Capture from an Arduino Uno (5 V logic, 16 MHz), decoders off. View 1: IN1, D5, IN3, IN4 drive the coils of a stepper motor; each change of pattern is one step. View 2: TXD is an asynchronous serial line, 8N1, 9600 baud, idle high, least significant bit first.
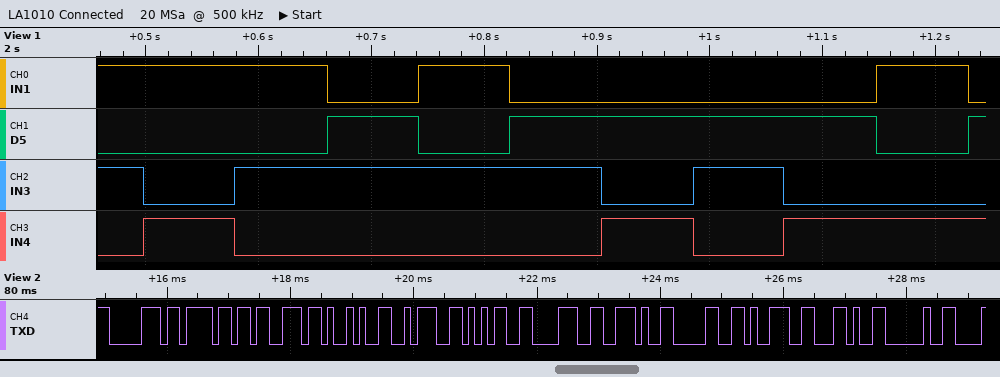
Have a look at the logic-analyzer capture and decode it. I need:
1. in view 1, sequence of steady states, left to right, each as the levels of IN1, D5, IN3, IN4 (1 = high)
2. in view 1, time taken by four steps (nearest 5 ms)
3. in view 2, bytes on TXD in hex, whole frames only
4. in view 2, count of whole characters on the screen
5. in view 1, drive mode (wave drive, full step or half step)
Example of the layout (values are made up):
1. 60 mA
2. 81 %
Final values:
1. 1010 1001 1010 0110 1010 0110 0101 0110 0101 1001 0101
2. 325 ms
3. 70 6F 73 29 3A 35 38 2E 30 39 2C 20
4. 12
5. full step
